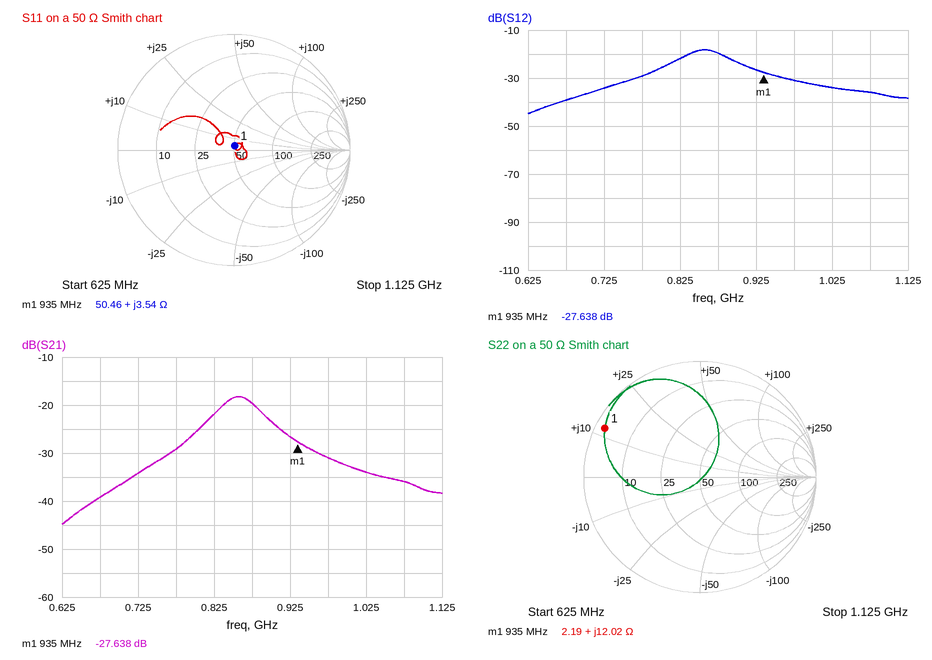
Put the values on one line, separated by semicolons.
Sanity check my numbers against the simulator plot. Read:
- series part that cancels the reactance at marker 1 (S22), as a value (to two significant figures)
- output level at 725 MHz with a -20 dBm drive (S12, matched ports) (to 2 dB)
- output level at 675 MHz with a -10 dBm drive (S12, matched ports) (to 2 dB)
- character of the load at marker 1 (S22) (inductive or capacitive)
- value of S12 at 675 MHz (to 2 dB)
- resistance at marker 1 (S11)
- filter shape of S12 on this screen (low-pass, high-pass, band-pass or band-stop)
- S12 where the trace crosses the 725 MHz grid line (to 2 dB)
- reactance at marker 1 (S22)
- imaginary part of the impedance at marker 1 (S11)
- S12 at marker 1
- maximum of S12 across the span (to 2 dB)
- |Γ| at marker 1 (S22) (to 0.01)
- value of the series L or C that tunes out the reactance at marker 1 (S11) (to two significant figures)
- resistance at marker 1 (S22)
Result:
14 pF; -54 dBm; -50 dBm; inductive; -40 dB; 50.46 Ω; band-pass; -34 dB; +12.02 Ω; +3.54 Ω; -27.638 dB; -18 dB; 0.92; 48 pF; 2.19 Ω
